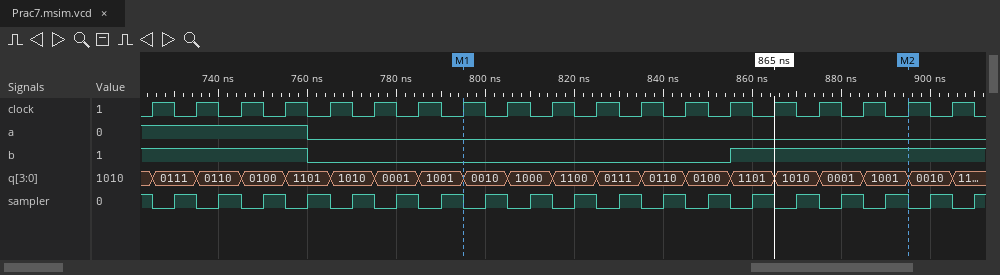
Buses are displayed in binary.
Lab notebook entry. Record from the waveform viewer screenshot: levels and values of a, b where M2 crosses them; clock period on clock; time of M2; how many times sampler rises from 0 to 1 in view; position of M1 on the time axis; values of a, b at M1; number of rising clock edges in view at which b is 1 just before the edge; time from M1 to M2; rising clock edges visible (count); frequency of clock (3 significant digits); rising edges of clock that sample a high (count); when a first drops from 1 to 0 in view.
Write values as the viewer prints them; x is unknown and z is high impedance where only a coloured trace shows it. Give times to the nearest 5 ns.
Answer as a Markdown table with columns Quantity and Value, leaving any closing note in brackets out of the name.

| Quantity | Value |
|---|---|
| levels and values of a, b where M2 crosses them | a=0, b=1 |
| clock period on clock | 10 ns |
| time of M2 | 895 ns |
| how many times sampler rises from 0 to 1 in view | 19 |
| position of M1 on the time axis | 795 ns |
| values of a, b at M1 | a=0, b=0 |
| number of rising clock edges in view at which b is 1 just before the edge | 9 |
| time from M1 to M2 | 100 ns |
| rising clock edges visible | 19 |
| frequency of clock | 100 MHz |
| rising edges of clock that sample a high | 4 |
| when a first drops from 1 to 0 in view | 760 ns |
